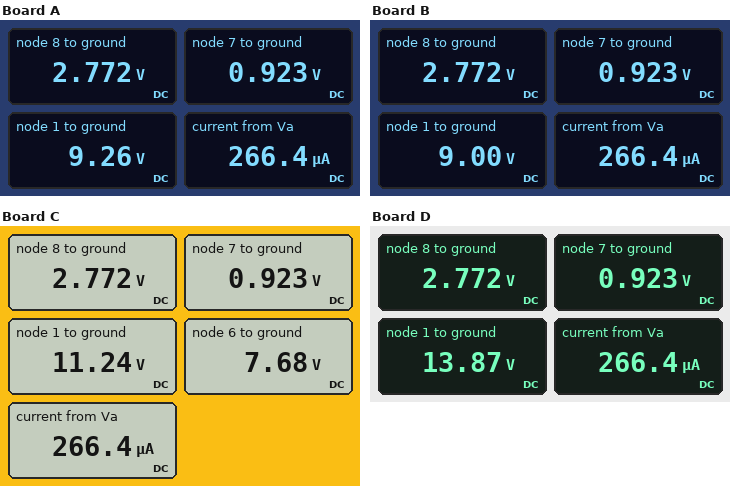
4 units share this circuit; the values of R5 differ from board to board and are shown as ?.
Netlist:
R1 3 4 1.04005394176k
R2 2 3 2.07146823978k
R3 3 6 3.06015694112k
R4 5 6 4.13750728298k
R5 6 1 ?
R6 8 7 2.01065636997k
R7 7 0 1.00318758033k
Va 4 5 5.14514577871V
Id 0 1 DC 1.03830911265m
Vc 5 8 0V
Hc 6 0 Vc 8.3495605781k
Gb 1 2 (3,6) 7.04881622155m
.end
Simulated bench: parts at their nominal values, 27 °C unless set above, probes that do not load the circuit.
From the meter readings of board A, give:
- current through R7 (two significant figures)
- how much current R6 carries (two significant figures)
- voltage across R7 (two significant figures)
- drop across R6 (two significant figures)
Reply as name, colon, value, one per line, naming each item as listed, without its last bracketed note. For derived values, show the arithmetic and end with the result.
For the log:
current through R7: (923 mV) / 1.003 kΩ = 920 µA
how much current R6 carries: (2.772 V - 923 mV) / 2.011 kΩ = 920 µA
voltage across R7: 923 mV = 920 mV
drop across R6: 2.772 V - 923 mV = 1.8 V
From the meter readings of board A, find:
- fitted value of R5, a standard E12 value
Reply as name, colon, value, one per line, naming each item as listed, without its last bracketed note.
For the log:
fitted value of R5, a standard E12 value: 1.2 kΩ
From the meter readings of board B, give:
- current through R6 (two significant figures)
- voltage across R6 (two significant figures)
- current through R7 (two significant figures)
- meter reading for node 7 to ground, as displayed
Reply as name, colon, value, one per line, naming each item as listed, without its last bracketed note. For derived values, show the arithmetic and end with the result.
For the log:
current through R6: (2.772 V - 923 mV) / 2.011 kΩ = 920 µA
voltage across R6: 2.772 V - 923 mV = 1.8 V
current through R7: (923 mV) / 1.003 kΩ = 920 µA
meter reading for node 7 to ground, as displayed: 0.923 V
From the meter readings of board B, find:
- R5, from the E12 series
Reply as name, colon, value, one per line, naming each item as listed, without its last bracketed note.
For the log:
R5, from the E12 series: 1 kΩ
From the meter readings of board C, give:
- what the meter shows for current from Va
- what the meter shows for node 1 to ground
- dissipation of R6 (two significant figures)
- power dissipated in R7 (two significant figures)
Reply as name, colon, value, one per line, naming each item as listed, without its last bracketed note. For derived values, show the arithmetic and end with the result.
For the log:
what the meter shows for current from Va: 266.4 µA
what the meter shows for node 1 to ground: 11.24 V
dissipation of R6: (2.772 V - 923 mV)^2 / 2.011 kΩ = 1.7 mW
power dissipated in R7: (923 mV)^2 / 1.003 kΩ = 850 µW
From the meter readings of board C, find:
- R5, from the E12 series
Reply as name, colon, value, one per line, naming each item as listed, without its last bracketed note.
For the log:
R5, from the E12 series: 2.7 kΩ
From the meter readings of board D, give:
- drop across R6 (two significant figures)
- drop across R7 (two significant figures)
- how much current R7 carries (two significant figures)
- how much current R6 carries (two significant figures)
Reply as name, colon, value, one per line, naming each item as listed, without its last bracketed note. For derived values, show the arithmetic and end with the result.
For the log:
drop across R6: 2.772 V - 923 mV = 1.8 V
drop across R7: 923 mV = 920 mV
how much current R7 carries: (923 mV) / 1.003 kΩ = 920 µA
how much current R6 carries: (2.772 V - 923 mV) / 2.011 kΩ = 920 µA
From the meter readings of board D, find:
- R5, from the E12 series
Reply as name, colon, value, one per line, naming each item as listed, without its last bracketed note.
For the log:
R5, from the E12 series: 4.7 kΩ
